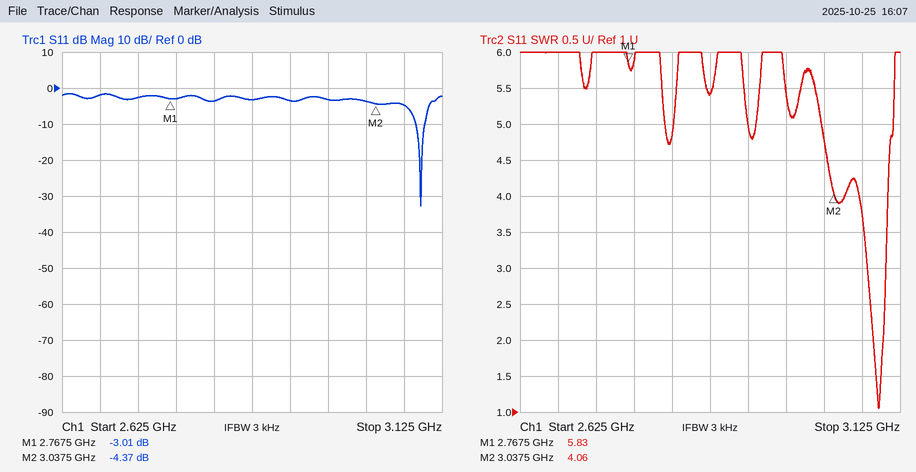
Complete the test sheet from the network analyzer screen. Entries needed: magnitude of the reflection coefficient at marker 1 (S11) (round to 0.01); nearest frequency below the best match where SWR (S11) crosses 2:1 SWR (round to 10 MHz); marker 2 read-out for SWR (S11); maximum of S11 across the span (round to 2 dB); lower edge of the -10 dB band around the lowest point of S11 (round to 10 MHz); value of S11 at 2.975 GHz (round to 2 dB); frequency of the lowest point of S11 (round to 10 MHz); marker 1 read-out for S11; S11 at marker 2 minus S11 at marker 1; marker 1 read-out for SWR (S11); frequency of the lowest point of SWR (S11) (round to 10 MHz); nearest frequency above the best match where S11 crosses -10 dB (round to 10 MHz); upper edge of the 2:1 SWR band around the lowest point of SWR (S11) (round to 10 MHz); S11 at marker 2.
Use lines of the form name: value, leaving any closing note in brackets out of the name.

magnitude of the reflection coefficient at marker 1 (S11): 0.71
nearest frequency below the best match where SWR (S11) crosses 2:1 SWR: 3.09 GHz
marker 2 read-out for SWR: 4.06
maximum of S11 across the span: -2 dB
lower edge of the -10 dB band around the lowest point of S11: 3.09 GHz
value of S11 at 2.975 GHz: -4 dB
frequency of the lowest point of S11: 3.10 GHz
marker 1 read-out for S11: -3.01 dB
S11 at marker 2 minus S11 at marker 1: -1.36 dB
marker 1 read-out for SWR: 5.83
frequency of the lowest point of SWR (S11): 3.10 GHz
nearest frequency above the best match where S11 crosses -10 dB: 3.10 GHz
upper edge of the 2:1 SWR band around the lowest point of SWR (S11): 3.10 GHz
S11 at marker 2: -4.37 dB
